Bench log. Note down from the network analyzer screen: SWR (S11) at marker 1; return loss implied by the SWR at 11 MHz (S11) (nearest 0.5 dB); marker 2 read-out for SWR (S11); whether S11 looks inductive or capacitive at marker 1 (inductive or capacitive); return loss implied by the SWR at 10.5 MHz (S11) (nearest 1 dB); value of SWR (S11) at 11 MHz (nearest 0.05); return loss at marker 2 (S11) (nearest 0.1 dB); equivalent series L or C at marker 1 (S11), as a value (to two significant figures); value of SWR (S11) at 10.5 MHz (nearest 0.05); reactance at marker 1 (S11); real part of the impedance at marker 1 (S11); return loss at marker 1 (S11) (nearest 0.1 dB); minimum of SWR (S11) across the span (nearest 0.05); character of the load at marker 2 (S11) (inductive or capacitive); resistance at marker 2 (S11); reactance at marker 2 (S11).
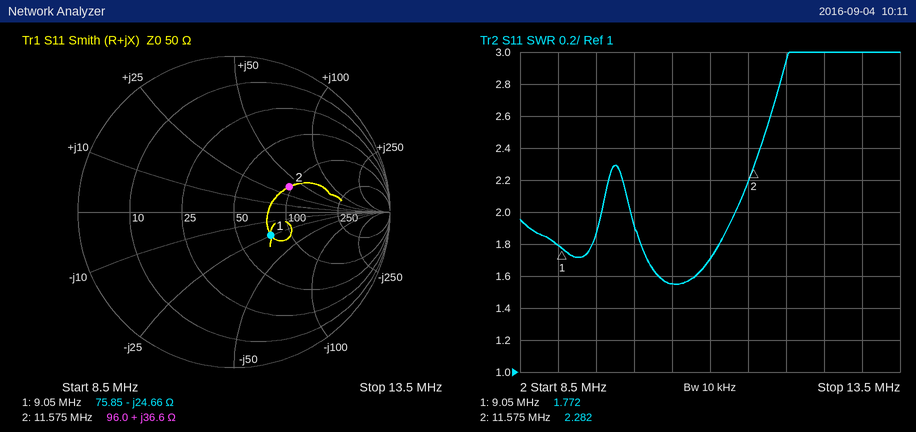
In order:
1.772
11.5 dB
2.282
capacitive
13 dB
1.70
8.2 dB
710 pF
1.55
-24.66 Ω
75.85 Ω
11.1 dB
1.55
inductive
96.0 Ω
+36.6 Ω
